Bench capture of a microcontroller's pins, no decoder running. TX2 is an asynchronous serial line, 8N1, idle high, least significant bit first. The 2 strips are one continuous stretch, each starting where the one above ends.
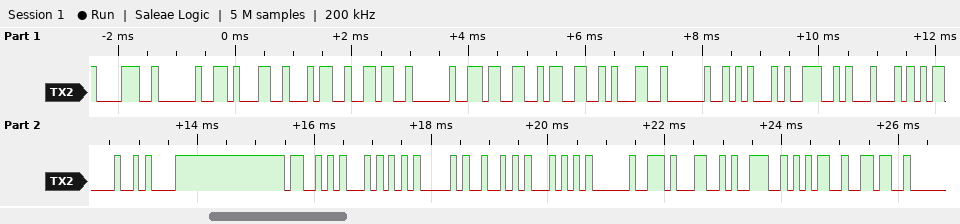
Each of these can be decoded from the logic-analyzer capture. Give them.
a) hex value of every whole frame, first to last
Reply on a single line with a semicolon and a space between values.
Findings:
38 20 31 34 36 20 33 33 31 20 45 4E 44 0D 0A 53 54 41 52 54 20 31 39 35 36
